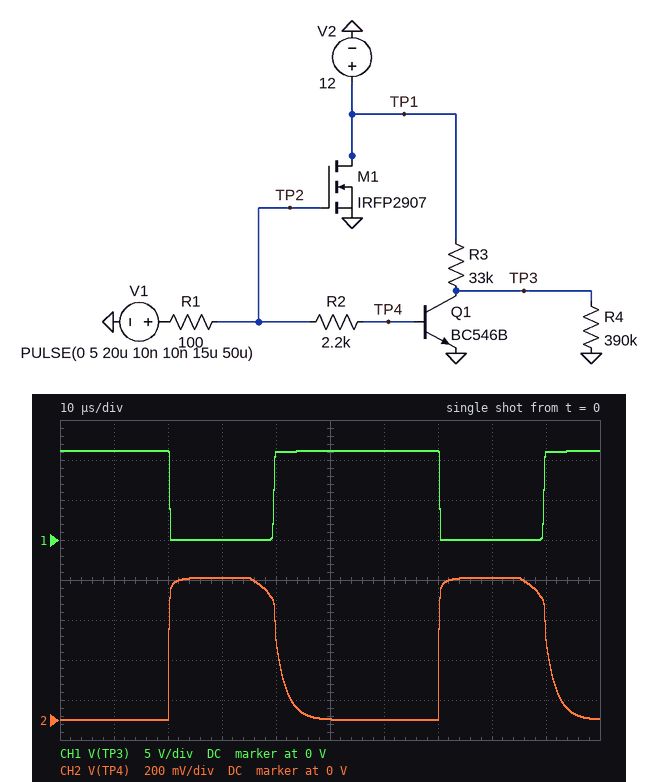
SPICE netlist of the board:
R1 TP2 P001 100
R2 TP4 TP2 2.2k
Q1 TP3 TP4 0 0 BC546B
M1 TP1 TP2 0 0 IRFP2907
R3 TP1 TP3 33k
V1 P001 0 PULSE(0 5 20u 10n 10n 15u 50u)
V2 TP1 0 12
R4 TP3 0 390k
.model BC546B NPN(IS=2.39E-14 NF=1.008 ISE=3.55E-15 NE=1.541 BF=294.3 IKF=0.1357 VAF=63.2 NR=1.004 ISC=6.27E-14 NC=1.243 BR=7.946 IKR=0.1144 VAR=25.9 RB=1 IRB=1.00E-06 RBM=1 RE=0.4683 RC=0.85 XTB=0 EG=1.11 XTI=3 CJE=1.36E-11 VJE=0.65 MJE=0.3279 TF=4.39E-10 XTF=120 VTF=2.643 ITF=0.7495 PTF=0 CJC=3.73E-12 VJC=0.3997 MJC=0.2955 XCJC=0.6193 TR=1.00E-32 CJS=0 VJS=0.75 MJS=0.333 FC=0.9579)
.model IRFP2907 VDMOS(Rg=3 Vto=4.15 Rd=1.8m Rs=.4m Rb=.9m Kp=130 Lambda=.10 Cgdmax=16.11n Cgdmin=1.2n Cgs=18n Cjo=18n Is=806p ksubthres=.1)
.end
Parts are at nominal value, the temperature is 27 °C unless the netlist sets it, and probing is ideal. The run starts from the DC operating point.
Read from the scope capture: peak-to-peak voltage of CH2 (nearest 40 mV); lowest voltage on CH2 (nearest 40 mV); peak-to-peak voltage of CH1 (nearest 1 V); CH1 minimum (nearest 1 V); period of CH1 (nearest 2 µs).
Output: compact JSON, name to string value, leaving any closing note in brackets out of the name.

{"peak-to-peak voltage of CH2": "720 mV", "lowest voltage on CH2": "0 V", "peak-to-peak voltage of CH1": "11 V", "CH1 minimum": "0 V", "period of CH1": "50 µs"}
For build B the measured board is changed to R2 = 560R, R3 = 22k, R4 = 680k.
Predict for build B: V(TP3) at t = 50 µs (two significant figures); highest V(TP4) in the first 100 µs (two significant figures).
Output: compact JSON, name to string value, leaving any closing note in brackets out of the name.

{"V(TP3) at t = 50 µs": "12 V", "highest V(TP4) in the first 100 µs": "750 mV"}
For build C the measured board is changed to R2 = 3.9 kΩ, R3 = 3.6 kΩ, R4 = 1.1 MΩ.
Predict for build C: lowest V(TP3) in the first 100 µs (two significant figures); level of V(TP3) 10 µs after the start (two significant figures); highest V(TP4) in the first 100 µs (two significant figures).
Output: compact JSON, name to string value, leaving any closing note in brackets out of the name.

{"lowest V(TP3) in the first 100 µs": "22 mV", "level of V(TP3) 10 µs after the start": "12 V", "highest V(TP4) in the first 100 µs": "710 mV"}
